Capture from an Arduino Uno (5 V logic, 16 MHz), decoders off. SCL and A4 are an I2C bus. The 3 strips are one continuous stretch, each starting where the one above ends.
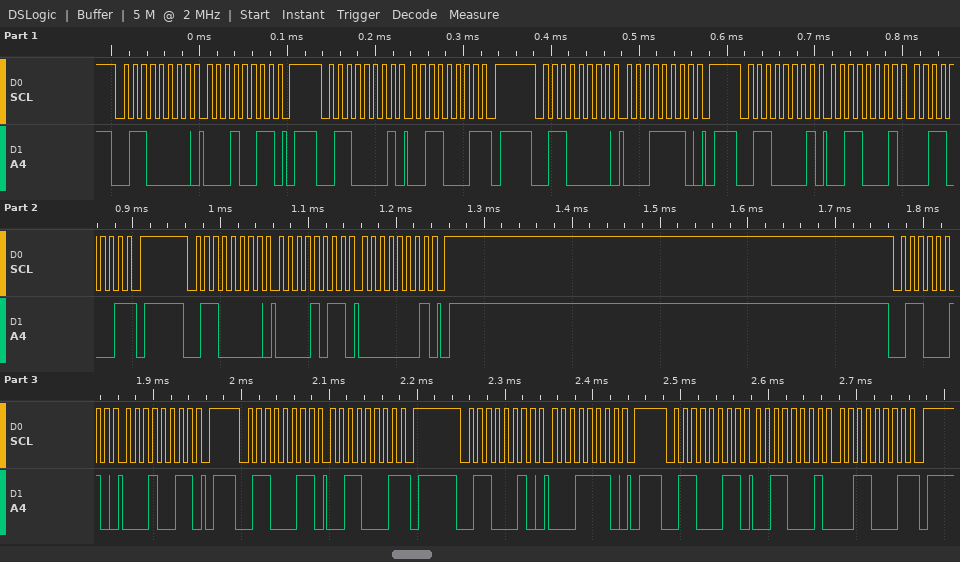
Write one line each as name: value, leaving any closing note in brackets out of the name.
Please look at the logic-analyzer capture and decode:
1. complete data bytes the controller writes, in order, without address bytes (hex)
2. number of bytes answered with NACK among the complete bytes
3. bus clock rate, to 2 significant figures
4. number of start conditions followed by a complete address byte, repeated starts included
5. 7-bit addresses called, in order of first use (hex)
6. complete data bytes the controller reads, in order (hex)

complete data bytes the controller writes, in order, without address bytes: 13 1E 0B 01 13 1E
number of bytes answered with NACK among the complete bytes: 4
bus clock rate, to 2 significant figures: 100 kHz
number of start conditions followed by a complete address byte, repeated starts included: 9
7-bit addresses called, in order of first use: 0x30 0x31
complete data bytes the controller reads, in order: 31 31 31 31 31 31
